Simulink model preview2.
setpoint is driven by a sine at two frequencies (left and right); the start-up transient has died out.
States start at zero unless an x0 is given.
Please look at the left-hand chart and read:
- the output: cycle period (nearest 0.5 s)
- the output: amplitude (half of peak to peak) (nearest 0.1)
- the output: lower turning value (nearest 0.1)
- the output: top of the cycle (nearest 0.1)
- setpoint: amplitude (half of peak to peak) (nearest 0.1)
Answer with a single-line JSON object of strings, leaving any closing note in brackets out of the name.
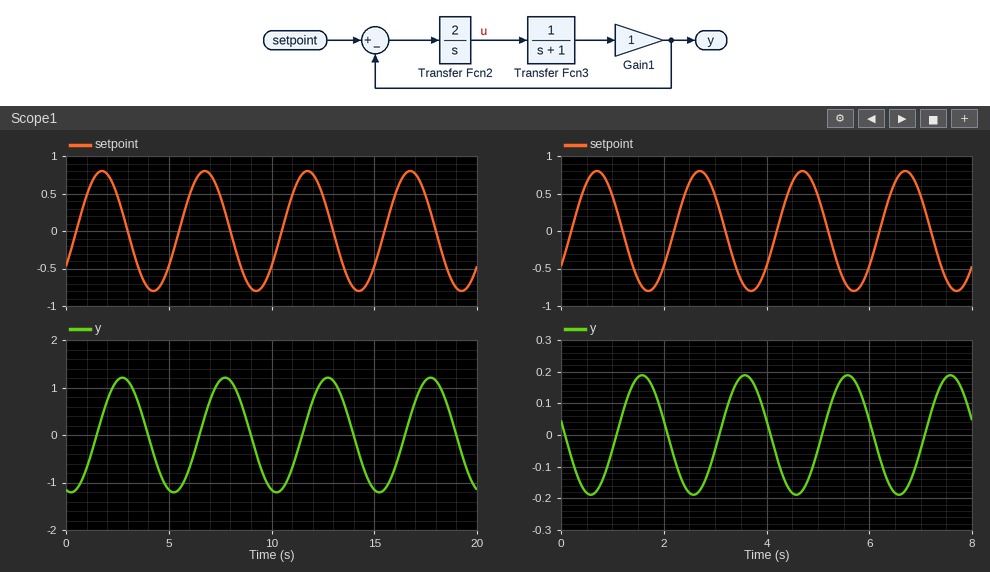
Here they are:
{"the output: cycle period": "5.0 s", "the output: amplitude (half of peak to peak)": "1.2", "the output: lower turning value": "-1.2", "the output: top of the cycle": "1.2", "setpoint: amplitude (half of peak to peak)": "0.8"}
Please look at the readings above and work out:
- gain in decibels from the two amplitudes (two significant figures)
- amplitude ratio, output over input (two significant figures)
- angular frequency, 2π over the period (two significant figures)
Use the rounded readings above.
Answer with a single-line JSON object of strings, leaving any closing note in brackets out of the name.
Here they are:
{"gain in decibels from the two amplitudes": "3.5 dB", "amplitude ratio, output over input": "1.5", "angular frequency, 2π over the period": "1.3 rad/s"}
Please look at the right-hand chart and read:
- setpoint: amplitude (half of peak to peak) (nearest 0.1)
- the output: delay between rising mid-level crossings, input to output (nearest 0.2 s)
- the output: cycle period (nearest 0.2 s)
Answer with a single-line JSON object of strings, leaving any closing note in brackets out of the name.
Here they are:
{"setpoint: amplitude (half of peak to peak)": "0.8", "the output: delay between rising mid-level crossings, input to output": "0.8 s", "the output: cycle period": "2.0 s"}
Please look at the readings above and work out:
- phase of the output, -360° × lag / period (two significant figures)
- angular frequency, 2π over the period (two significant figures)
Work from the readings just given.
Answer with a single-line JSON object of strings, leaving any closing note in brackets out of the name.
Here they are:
{"phase of the output, -360° × lag / period": "-140°", "angular frequency, 2π over the period": "3.1 rad/s"}
